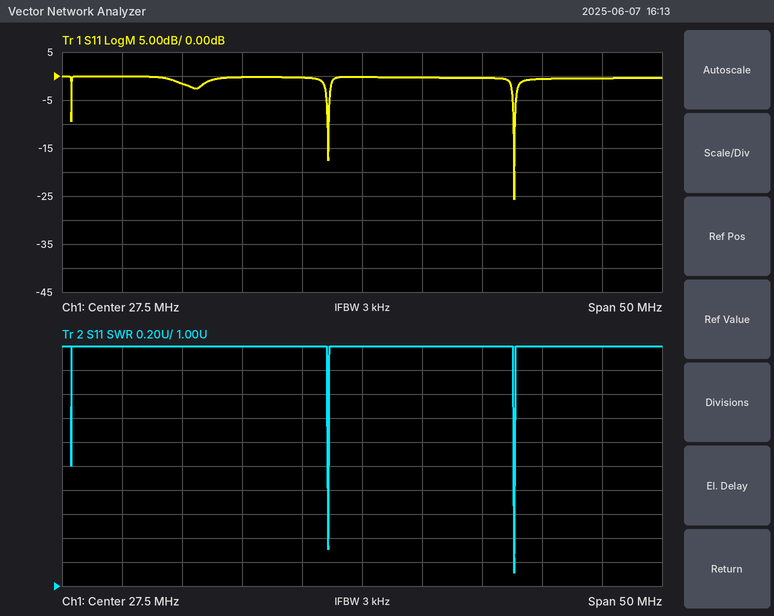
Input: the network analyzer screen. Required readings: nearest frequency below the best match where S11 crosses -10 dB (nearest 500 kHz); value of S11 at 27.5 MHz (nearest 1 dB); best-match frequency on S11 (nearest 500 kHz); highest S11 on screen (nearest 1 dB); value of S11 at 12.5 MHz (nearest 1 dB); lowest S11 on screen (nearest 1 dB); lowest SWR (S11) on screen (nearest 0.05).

40.0 MHz
0 dB
40.0 MHz
0 dB
-2 dB
-26 dB
1.10
